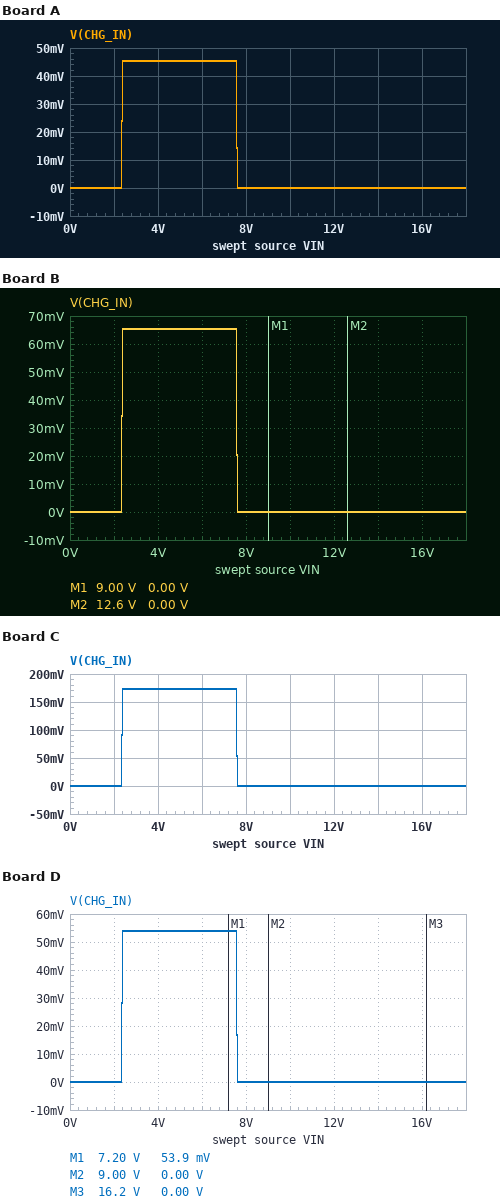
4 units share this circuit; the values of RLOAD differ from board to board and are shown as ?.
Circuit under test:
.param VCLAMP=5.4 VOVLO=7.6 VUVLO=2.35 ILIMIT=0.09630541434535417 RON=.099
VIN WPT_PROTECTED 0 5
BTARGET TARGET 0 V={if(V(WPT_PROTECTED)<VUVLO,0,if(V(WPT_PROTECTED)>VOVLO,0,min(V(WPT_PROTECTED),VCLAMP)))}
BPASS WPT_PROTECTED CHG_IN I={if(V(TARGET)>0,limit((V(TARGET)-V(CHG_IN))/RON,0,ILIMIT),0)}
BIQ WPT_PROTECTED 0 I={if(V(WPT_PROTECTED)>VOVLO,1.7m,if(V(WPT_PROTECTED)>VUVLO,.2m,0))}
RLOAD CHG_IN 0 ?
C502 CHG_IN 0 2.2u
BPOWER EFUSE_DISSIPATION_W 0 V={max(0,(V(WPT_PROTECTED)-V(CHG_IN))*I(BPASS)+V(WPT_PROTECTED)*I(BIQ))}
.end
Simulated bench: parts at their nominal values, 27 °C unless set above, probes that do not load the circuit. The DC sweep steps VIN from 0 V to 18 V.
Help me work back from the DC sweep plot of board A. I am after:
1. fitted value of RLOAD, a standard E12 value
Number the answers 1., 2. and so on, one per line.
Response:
1. 0.47 Ω
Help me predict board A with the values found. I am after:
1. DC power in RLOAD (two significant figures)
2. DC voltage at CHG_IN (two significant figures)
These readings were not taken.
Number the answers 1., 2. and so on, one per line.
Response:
1. 4.4 mW
2. 45 mV
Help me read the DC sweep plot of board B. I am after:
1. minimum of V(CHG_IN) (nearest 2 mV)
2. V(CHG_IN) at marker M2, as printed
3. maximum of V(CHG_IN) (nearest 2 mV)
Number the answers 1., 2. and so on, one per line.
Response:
1. 0 V
2. 0.00 V
3. 66 mV
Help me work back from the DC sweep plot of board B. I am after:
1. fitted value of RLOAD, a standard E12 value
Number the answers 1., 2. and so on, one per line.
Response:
1. 0.68 Ω
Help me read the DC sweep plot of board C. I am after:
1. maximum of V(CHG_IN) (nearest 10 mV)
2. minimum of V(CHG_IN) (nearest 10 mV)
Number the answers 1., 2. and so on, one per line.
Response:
1. 170 mV
2. 0 V
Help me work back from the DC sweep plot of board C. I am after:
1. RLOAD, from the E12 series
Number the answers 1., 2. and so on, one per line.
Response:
1. 1.8 Ω
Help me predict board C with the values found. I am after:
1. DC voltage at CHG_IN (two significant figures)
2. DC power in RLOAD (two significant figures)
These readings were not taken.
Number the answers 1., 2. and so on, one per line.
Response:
1. 170 mV
2. 17 mW
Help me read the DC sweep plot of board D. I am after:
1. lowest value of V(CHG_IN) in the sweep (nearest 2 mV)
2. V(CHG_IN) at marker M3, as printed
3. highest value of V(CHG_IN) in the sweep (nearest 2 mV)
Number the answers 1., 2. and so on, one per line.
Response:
1. 0 V
2. 0.00 V
3. 54 mV
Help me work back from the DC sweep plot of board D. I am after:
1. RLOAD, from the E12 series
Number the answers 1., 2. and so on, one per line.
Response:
1. 0.56 Ω
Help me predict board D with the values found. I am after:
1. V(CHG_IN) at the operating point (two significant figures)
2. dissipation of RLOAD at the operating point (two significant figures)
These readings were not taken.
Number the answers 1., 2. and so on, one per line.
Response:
1. 54 mV
2. 5.2 mW
